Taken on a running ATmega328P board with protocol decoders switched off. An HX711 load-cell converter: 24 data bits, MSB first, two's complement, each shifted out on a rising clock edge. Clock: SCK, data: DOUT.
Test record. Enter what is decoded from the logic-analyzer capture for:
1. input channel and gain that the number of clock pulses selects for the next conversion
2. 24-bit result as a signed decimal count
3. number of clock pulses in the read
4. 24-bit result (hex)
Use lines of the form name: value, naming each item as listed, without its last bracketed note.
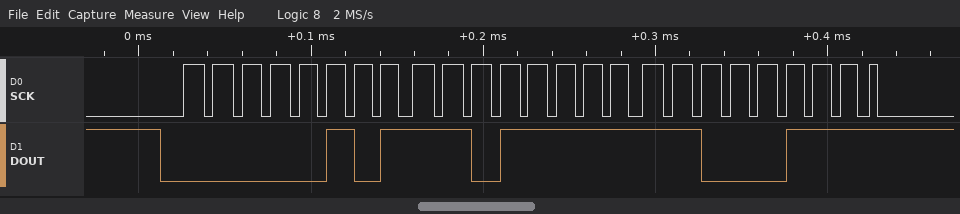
input channel and gain that the number of clock pulses selects for the next conversion: channel A, gain 128
24-bit result as a signed decimal count: 384967
number of clock pulses in the read: 25
24-bit result: 0x05DFC7
